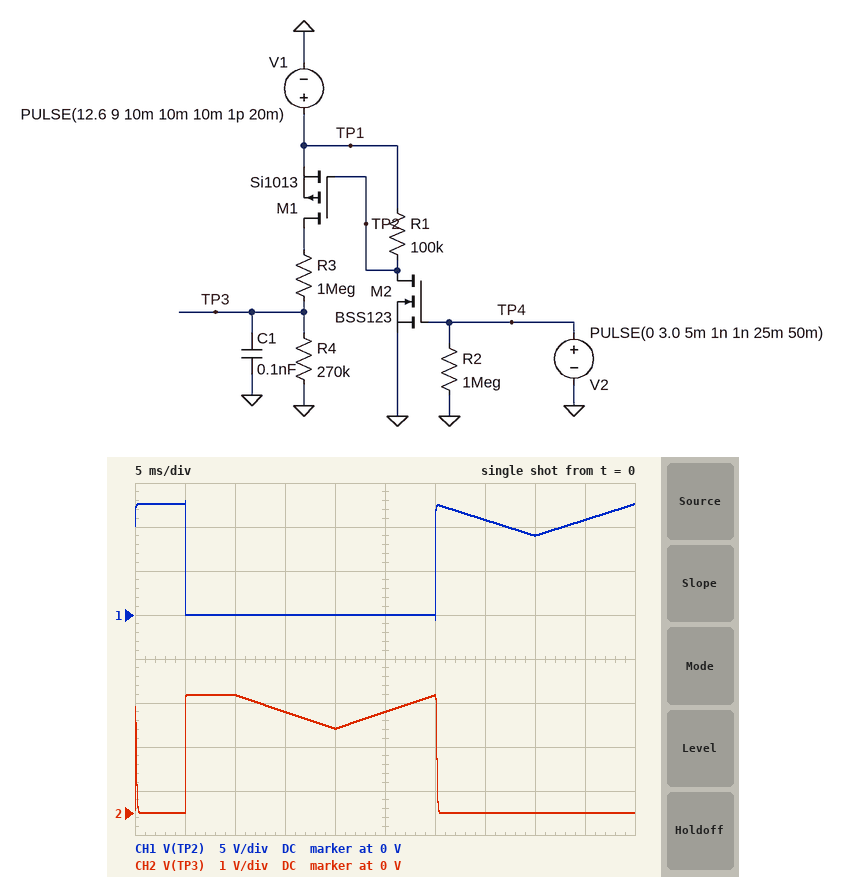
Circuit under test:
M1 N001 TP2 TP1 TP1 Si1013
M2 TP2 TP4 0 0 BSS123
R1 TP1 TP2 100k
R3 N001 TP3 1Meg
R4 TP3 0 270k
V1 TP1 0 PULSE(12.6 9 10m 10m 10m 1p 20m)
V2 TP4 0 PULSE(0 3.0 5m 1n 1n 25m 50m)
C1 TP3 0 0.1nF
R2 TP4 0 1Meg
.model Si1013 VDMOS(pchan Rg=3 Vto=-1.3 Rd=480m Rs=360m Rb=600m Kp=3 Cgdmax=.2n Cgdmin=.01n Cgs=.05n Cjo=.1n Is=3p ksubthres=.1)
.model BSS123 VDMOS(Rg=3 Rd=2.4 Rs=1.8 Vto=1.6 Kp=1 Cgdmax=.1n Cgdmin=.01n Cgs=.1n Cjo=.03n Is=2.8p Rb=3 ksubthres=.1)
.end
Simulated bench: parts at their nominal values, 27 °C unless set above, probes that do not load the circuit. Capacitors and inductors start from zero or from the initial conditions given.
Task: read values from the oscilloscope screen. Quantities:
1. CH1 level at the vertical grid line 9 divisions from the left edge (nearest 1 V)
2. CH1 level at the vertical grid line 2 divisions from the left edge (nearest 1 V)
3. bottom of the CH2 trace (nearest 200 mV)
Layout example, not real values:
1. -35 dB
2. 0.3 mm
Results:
1. 11 V
2. 0 V
3. 0 V
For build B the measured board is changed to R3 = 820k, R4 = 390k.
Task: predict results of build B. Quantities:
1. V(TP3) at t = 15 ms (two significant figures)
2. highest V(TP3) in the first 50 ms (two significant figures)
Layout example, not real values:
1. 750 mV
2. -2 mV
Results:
1. 3.5 V
2. 4.1 V
